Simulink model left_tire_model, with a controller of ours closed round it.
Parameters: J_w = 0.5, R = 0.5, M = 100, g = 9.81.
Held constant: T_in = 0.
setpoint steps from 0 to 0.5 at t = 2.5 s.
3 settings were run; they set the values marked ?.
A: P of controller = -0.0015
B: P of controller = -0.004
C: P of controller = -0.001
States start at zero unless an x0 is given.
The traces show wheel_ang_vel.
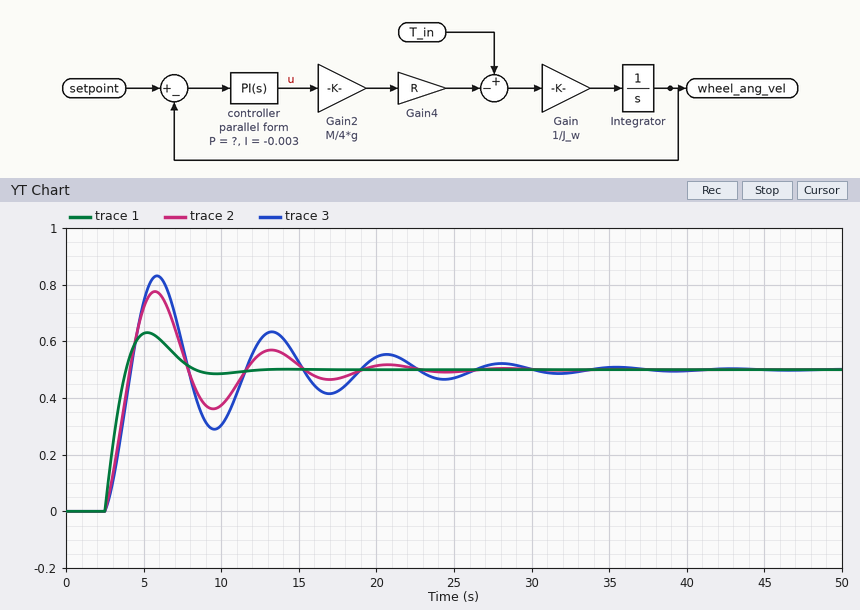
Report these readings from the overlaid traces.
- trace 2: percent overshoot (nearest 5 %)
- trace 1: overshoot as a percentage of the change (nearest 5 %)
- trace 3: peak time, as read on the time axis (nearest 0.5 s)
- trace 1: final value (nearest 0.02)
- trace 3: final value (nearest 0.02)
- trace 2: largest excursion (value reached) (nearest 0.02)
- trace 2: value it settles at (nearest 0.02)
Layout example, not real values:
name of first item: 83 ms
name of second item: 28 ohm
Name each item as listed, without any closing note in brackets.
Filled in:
trace 2: percent overshoot: 55 %
trace 1: overshoot as a percentage of the change: 25 %
trace 3: peak time, as read on the time axis: 6.0 s
trace 1: final value: 0.50
trace 3: final value: 0.50
trace 2: largest excursion (value reached): 0.78
trace 2: value it settles at: 0.50
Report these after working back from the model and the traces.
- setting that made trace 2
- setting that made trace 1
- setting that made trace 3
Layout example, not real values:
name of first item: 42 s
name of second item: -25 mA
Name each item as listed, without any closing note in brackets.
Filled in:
setting that made trace 2: A
setting that made trace 1: B
setting that made trace 3: C
